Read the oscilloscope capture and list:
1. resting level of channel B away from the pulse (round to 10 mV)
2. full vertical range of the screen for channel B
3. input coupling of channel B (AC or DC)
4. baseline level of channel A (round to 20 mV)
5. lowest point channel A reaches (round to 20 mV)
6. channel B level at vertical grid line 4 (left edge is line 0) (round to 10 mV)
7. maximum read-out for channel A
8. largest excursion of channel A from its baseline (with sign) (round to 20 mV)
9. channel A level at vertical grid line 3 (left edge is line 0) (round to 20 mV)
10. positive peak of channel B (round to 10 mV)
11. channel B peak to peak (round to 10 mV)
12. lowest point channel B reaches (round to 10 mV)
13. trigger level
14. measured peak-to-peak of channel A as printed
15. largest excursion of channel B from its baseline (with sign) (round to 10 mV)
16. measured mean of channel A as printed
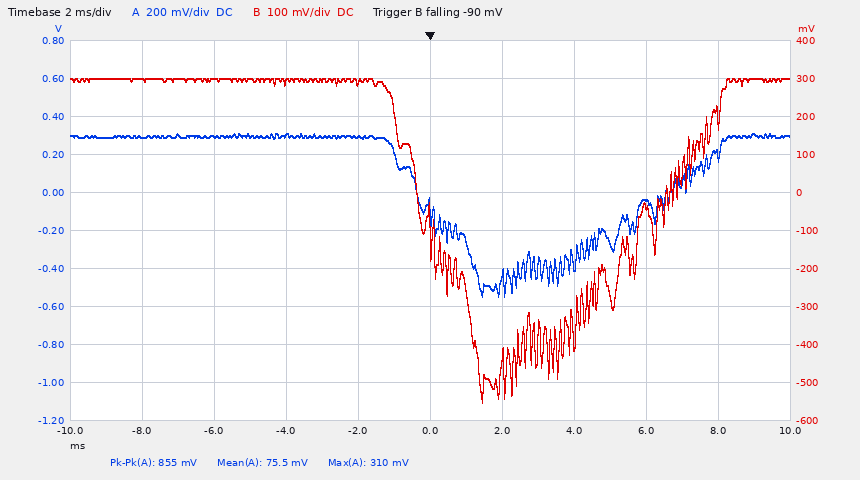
300 mV
1 V
DC
300 mV
-540 mV
290 mV
310 mV
-840 mV
300 mV
300 mV
850 mV
-550 mV
-90 mV
855 mV
-850 mV
75.5 mV
